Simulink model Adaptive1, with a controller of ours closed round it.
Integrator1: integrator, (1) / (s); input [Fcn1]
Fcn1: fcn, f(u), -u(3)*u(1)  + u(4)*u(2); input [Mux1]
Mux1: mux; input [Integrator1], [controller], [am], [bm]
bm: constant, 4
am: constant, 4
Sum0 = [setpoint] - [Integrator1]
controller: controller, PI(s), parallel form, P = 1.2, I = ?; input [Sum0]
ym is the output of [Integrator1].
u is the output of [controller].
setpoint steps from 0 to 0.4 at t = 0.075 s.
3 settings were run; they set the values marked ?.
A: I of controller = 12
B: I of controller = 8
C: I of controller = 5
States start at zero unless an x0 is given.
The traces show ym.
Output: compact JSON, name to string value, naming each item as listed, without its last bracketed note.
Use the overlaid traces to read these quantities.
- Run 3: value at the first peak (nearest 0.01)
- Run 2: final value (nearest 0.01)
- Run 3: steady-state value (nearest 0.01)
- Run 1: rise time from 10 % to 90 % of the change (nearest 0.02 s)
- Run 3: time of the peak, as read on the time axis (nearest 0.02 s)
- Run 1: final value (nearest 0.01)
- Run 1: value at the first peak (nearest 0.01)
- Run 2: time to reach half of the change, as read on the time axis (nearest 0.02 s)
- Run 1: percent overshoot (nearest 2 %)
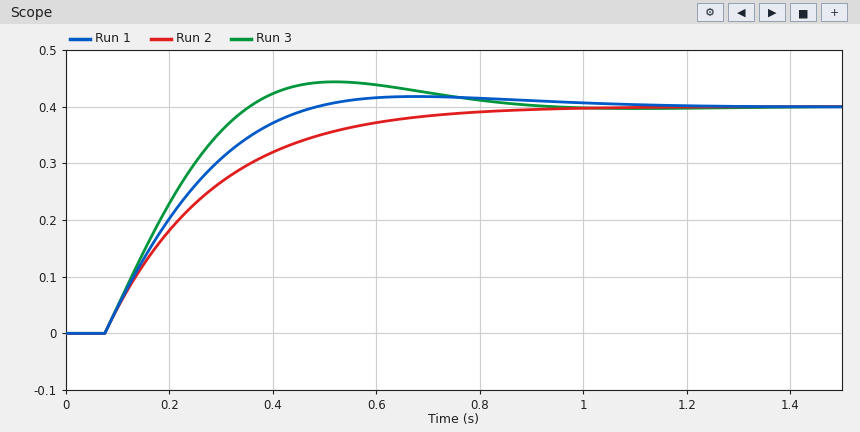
{"Run 3: value at the first peak": "0.44", "Run 2: final value": "0.40", "Run 3: steady-state value": "0.40", "Run 1: rise time from 10 % to 90 % of the change": "0.28 s", "Run 3: time of the peak, as read on the time axis": "0.52 s", "Run 1: final value": "0.40", "Run 1: value at the first peak": "0.42", "Run 2: time to reach half of the change, as read on the time axis": "0.22 s", "Run 1: percent overshoot": "4 %"}
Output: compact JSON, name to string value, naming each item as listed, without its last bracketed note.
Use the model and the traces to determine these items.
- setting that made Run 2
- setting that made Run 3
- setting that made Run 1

{"setting that made Run 2": "C", "setting that made Run 3": "A", "setting that made Run 1": "B"}
